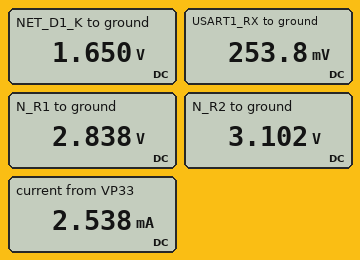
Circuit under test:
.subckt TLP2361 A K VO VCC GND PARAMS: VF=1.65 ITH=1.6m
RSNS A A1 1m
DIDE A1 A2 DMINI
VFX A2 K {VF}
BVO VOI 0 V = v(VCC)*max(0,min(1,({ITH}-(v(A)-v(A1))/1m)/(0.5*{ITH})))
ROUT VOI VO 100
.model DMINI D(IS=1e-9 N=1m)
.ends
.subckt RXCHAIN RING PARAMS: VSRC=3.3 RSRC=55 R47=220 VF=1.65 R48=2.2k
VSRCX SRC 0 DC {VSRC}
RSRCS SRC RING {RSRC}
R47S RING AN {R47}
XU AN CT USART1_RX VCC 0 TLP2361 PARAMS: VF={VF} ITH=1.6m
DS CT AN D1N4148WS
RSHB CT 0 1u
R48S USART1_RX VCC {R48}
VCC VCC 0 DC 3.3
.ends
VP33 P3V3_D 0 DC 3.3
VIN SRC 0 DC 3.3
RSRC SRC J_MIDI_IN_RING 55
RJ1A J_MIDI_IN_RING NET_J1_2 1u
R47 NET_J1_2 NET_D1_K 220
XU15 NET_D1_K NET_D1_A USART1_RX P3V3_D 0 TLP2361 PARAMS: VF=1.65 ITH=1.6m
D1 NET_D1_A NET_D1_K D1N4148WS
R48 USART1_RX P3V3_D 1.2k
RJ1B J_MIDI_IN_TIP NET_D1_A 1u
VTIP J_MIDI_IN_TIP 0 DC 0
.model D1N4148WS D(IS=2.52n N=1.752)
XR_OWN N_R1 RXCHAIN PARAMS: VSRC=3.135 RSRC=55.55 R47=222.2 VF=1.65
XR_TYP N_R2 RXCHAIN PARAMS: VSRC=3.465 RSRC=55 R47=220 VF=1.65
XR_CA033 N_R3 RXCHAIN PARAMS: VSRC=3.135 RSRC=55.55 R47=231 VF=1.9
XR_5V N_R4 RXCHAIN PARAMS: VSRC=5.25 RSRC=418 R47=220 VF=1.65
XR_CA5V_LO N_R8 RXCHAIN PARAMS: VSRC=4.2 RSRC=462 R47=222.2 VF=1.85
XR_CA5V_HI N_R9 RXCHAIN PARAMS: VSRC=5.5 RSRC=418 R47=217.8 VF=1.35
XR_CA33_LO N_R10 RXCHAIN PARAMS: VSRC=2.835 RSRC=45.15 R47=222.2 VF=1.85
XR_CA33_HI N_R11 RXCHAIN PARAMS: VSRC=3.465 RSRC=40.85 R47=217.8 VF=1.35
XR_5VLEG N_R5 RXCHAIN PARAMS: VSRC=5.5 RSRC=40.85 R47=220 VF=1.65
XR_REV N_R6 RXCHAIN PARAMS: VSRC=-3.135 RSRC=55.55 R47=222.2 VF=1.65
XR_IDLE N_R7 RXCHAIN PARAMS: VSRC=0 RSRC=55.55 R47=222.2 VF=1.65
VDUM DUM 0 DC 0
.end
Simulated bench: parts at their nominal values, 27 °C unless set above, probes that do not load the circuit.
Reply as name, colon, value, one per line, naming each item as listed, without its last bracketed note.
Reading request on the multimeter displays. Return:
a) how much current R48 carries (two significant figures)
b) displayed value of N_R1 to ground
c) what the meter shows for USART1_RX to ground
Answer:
how much current R48 carries: 2.5 mA
displayed value of N_R1 to ground: 2.838 V
what the meter shows for USART1_RX to ground: 253.8 mV
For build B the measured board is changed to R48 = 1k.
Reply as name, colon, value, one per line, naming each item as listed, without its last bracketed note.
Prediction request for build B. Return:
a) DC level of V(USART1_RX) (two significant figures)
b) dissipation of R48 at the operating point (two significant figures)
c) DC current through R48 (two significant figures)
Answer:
DC level of V(USART1_RX): 300 mV
dissipation of R48 at the operating point: 9.0 mW
DC current through R48: 3.0 mA
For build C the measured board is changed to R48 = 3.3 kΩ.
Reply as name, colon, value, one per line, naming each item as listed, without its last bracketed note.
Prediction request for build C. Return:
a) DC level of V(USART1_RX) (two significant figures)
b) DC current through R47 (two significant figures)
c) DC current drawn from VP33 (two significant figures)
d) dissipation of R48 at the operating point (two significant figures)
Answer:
DC level of V(USART1_RX): 97 mV
DC current through R47: 6.0 mA
DC current drawn from VP33: 970 µA
dissipation of R48 at the operating point: 3.1 mW
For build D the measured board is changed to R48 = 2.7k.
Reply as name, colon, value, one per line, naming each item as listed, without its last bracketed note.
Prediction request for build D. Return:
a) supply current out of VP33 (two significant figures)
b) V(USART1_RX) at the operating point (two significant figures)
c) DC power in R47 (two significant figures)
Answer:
supply current out of VP33: 1.2 mA
V(USART1_RX) at the operating point: 120 mV
DC power in R47: 7.9 mW
